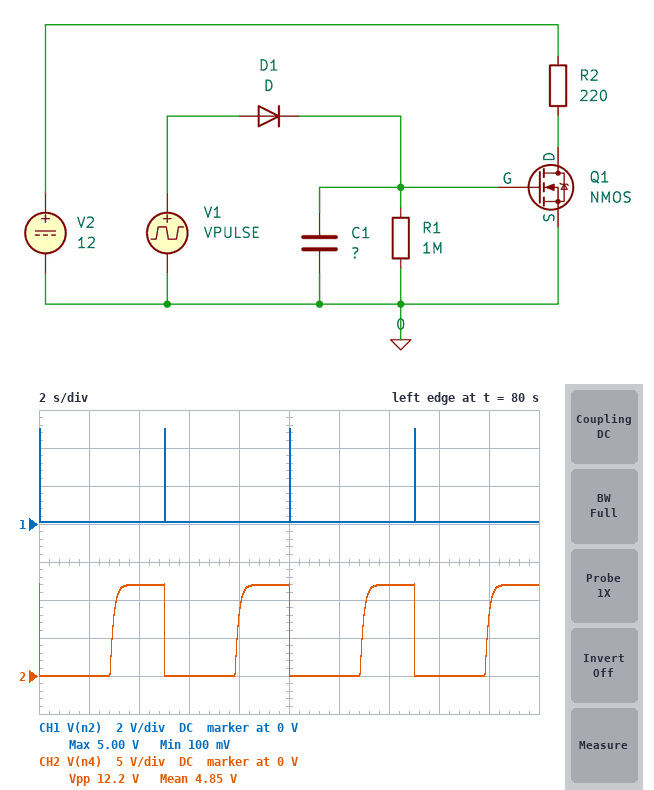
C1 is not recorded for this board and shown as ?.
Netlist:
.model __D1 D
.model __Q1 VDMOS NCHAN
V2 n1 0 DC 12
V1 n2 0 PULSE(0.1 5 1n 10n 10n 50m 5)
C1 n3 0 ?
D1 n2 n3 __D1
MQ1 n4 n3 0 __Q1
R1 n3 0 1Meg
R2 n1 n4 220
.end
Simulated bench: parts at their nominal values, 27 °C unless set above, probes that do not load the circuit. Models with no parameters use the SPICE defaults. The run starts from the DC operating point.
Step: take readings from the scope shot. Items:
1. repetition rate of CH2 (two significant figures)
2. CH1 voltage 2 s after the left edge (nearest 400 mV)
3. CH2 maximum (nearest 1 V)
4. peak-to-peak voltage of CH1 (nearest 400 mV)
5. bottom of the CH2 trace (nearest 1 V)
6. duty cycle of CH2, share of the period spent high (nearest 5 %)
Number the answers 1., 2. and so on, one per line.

1. 200 mHz
2. 0 V
3. 12 V
4. 4.8 V
5. 0 V
6. 40 %
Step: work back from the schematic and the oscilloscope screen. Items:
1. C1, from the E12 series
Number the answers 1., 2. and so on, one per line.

1. 6.8 µF
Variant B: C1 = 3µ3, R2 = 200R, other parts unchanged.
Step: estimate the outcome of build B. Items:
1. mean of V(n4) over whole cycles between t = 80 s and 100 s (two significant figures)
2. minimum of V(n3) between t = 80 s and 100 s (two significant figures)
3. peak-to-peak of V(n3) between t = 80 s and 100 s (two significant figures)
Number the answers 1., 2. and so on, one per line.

1. 8.5 V
2. 1.0 V
3. 3.5 V
